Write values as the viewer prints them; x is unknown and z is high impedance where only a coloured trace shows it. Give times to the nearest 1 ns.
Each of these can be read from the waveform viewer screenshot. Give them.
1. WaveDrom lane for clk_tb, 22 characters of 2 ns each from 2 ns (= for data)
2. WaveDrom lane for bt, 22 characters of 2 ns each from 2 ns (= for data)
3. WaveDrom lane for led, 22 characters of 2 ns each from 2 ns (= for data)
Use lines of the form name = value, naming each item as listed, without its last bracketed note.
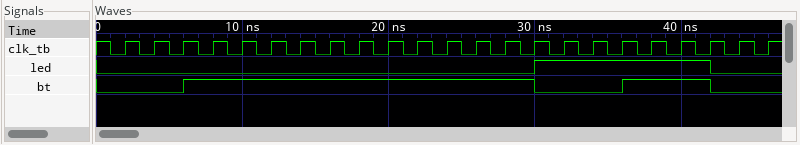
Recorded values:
WaveDrom lane for clk_tb, 22 characters of 2 ns each from 2 ns = {name: 'clk_tb', wave: 'p.....................'}
WaveDrom lane for bt, 22 characters of 2 ns each from 2 ns = {name: 'bt', wave: '0.1...........0..1..0.'}
WaveDrom lane for led, 22 characters of 2 ns each from 2 ns = {name: 'led', wave: '0.............1.....0.'}
